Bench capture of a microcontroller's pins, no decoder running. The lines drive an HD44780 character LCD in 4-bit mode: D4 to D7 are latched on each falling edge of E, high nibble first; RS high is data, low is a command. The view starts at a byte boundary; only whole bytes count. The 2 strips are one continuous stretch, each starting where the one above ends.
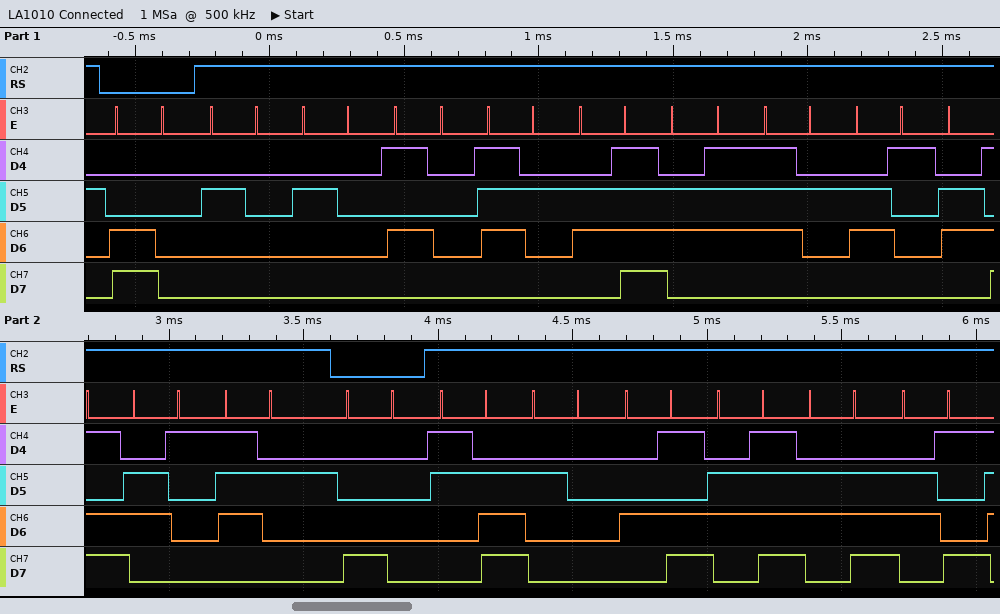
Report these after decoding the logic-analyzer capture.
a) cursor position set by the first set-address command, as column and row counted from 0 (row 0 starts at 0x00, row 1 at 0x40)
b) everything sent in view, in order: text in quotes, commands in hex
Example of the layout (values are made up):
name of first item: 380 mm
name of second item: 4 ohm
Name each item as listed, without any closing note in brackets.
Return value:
cursor position set by the first set-address command, as column and row counted from 0: column 0, row 1
everything sent in view, in order: text in quotes, commands in hex: 0xC0 "  Programar" 0x80 "> Moni"
